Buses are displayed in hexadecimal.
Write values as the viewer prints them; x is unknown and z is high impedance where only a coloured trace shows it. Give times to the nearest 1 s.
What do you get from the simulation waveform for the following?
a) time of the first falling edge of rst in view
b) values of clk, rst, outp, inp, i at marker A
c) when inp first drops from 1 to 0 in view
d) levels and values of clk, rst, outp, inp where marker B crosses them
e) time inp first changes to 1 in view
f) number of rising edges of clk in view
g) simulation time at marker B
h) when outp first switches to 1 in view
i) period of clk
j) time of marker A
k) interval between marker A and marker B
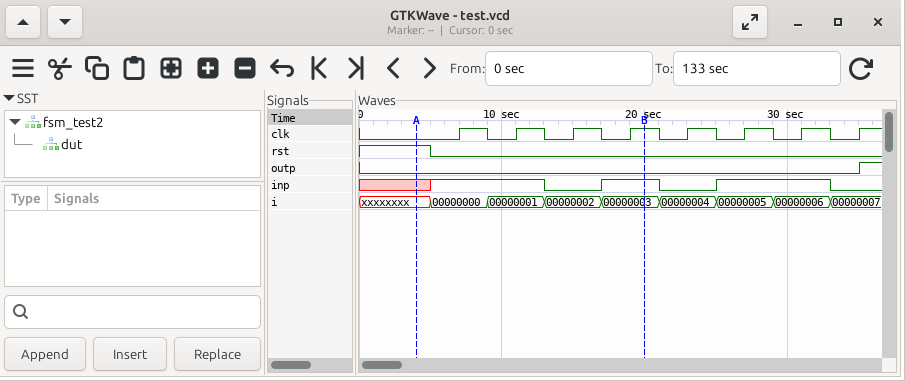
5 s
clk=0, rst=1, outp=0, inp=x, i=xxxxxxxx
13 s
clk=1, rst=0, outp=0, inp=1
5 s
8
20 s
35 s
4 s
4 s
16 s
